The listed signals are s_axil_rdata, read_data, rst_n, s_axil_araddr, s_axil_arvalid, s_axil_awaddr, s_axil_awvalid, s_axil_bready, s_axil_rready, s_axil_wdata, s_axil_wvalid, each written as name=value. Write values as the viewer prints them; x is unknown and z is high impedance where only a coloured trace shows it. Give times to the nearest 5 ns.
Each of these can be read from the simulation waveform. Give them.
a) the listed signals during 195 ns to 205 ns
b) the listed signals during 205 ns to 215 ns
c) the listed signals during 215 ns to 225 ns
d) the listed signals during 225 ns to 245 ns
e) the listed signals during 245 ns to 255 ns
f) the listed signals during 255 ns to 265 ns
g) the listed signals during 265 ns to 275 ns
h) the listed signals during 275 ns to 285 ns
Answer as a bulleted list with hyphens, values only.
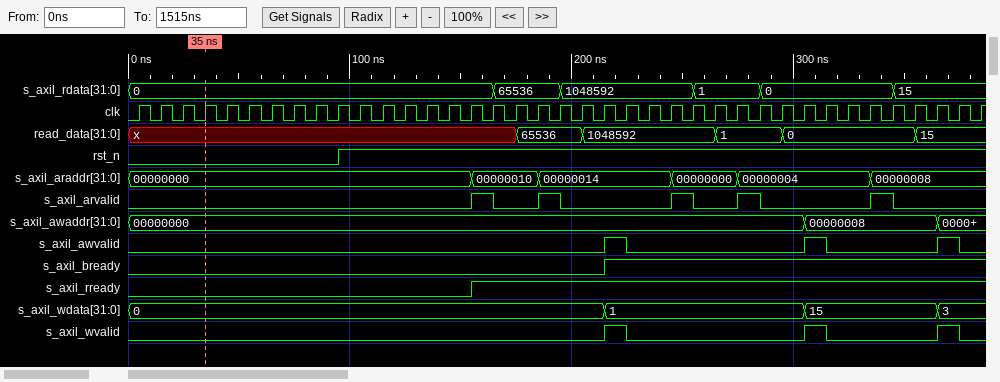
- s_axil_rdata=1048592, read_data=65536, rst_n=1, s_axil_araddr=00000014, s_axil_arvalid=0, s_axil_awaddr=00000000, s_axil_awvalid=0, s_axil_bready=0, s_axil_rready=1, s_axil_wdata=0, s_axil_wvalid=0
- s_axil_rdata=1048592, read_data=1048592, rst_n=1, s_axil_araddr=00000014, s_axil_arvalid=0, s_axil_awaddr=00000000, s_axil_awvalid=0, s_axil_bready=0, s_axil_rready=1, s_axil_wdata=0, s_axil_wvalid=0
- s_axil_rdata=1048592, read_data=1048592, rst_n=1, s_axil_araddr=00000014, s_axil_arvalid=0, s_axil_awaddr=00000000, s_axil_awvalid=1, s_axil_bready=1, s_axil_rready=1, s_axil_wdata=1, s_axil_wvalid=1
- s_axil_rdata=1048592, read_data=1048592, rst_n=1, s_axil_araddr=00000014, s_axil_arvalid=0, s_axil_awaddr=00000000, s_axil_awvalid=0, s_axil_bready=1, s_axil_rready=1, s_axil_wdata=1, s_axil_wvalid=0
- s_axil_rdata=1048592, read_data=1048592, rst_n=1, s_axil_araddr=00000000, s_axil_arvalid=1, s_axil_awaddr=00000000, s_axil_awvalid=0, s_axil_bready=1, s_axil_rready=1, s_axil_wdata=1, s_axil_wvalid=0
- s_axil_rdata=1, read_data=1048592, rst_n=1, s_axil_araddr=00000000, s_axil_arvalid=0, s_axil_awaddr=00000000, s_axil_awvalid=0, s_axil_bready=1, s_axil_rready=1, s_axil_wdata=1, s_axil_wvalid=0
- s_axil_rdata=1, read_data=1, rst_n=1, s_axil_araddr=00000000, s_axil_arvalid=0, s_axil_awaddr=00000000, s_axil_awvalid=0, s_axil_bready=1, s_axil_rready=1, s_axil_wdata=1, s_axil_wvalid=0
- s_axil_rdata=1, read_data=1, rst_n=1, s_axil_araddr=00000004, s_axil_arvalid=1, s_axil_awaddr=00000000, s_axil_awvalid=0, s_axil_bready=1, s_axil_rready=1, s_axil_wdata=1, s_axil_wvalid=0
